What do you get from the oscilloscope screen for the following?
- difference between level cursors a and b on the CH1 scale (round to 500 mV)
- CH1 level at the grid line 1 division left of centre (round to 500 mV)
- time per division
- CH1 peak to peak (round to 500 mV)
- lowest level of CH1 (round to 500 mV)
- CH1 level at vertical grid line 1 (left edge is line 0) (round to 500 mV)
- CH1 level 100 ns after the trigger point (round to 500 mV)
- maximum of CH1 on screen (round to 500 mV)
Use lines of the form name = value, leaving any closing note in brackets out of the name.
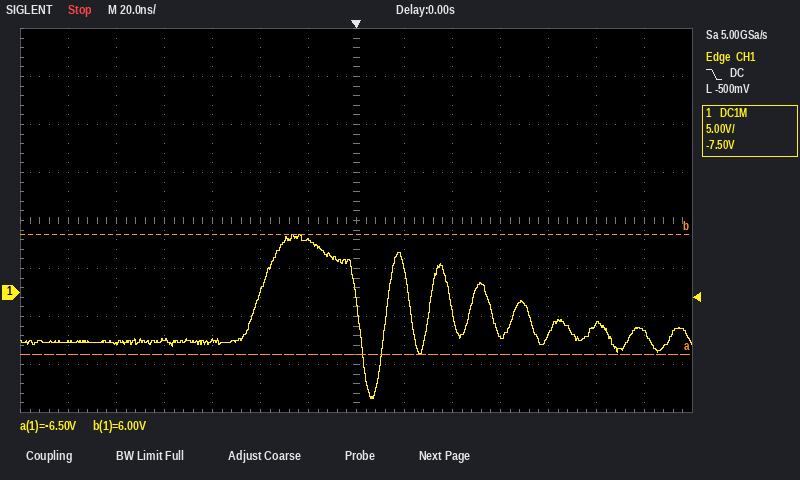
difference between level cursors a and b on the CH1 scale = 12.5 V
CH1 level at the grid line 1 division left of centre = 5.5 V
time per division = 20 ns
CH1 peak to peak = 17.0 V
lowest level of CH1 = -11.0 V
CH1 level at vertical grid line 1 (left edge is line 0) = -5.0 V
CH1 level 100 ns after the trigger point = -3.5 V
maximum of CH1 on screen = 6.0 V
